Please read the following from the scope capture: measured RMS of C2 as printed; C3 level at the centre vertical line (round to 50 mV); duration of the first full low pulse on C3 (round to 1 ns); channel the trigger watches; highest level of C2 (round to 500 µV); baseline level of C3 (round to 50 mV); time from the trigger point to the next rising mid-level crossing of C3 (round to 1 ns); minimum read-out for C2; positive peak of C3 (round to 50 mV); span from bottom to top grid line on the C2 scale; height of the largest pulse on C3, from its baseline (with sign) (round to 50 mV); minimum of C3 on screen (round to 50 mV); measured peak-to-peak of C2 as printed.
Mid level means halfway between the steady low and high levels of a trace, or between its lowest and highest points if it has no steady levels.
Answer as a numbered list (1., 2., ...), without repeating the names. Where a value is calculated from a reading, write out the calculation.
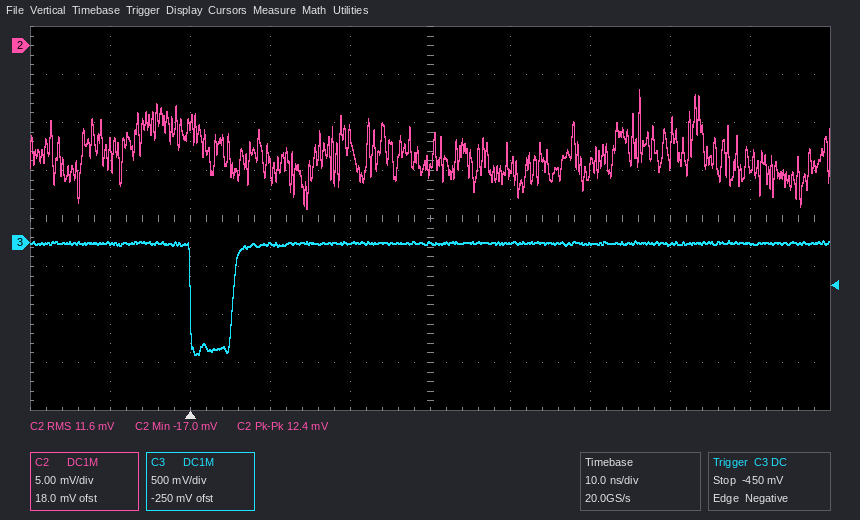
1. 11.6 mV
2. 0 mV
3. 5 ns
4. C3
5. -4.5 mV
6. 0 mV
7. 5 ns
8. -17.0 mV
9. 0 mV
10. 40 mV
11. -1.15 V − (0 mV) = -1.15 V
12. -1.15 V
13. 12.4 mV
